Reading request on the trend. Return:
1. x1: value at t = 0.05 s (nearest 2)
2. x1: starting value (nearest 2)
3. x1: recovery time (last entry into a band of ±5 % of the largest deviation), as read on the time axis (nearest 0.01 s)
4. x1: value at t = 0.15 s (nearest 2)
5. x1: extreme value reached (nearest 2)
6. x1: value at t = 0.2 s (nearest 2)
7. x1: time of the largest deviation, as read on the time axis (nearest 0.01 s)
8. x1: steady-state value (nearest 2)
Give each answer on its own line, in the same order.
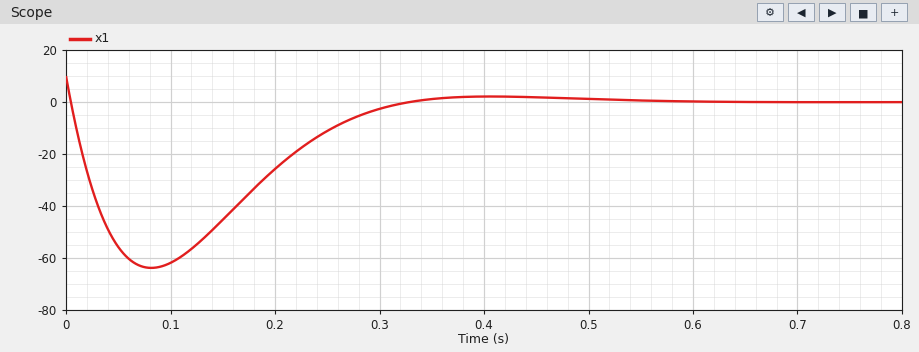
-56
10
0.29 s
-46
-64
-26
0.08 s
0
